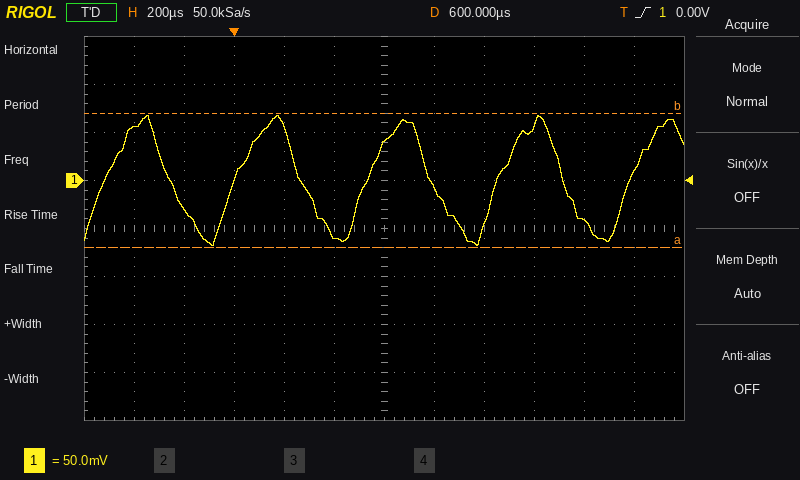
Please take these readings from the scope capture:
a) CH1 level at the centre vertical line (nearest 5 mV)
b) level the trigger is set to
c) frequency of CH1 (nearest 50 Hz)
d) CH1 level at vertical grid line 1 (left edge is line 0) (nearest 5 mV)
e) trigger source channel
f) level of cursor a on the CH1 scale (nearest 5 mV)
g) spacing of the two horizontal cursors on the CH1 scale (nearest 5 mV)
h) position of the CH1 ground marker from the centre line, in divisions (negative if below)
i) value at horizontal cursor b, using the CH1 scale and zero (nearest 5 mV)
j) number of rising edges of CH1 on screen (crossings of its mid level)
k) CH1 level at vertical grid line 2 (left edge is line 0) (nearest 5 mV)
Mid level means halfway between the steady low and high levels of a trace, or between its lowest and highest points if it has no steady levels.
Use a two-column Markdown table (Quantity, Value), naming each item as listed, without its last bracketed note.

| Quantity | Value |
|---|---|
| CH1 level at the centre vertical line | 40 mV |
| level the trigger is set to | 0.00 V |
| frequency of CH1 | 1.90 kHz |
| CH1 level at vertical grid line 1 (left edge is line 0) | 55 mV |
| trigger source channel | CH1 |
| level of cursor a on the CH1 scale | -70 mV |
| spacing of the two horizontal cursors on the CH1 scale | 140 mV |
| position of the CH1 ground marker from the centre line, in divisions | +1.0 div |
| value at horizontal cursor b, using the CH1 scale and zero | 70 mV |
| number of rising edges of CH1 on screen | 5 |
| CH1 level at vertical grid line 2 (left edge is line 0) | -30 mV |
